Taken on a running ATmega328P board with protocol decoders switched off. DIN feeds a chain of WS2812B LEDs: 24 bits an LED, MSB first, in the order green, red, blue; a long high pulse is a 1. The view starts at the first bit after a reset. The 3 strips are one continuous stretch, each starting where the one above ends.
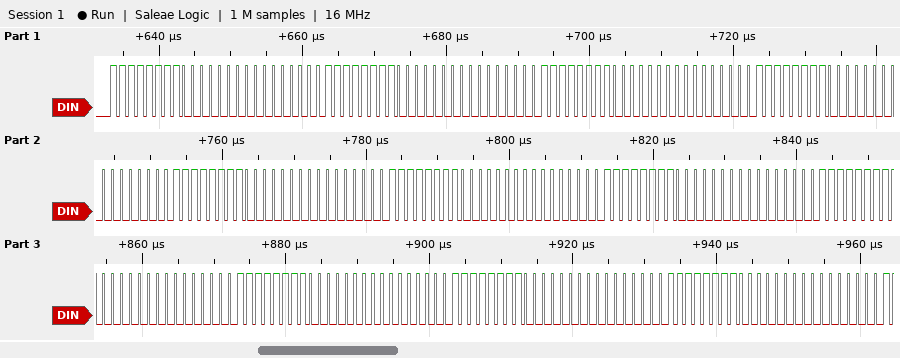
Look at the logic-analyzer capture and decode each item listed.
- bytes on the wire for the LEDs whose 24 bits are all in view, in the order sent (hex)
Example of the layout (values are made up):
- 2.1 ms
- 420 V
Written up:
- FF 00 00 FF 00 00 FF 00 00 FF 00 00 FF 00 00 FF 00 00 FF 00 00 FF 00 00 FF 00 00 FF 00 00 FF 00 00
